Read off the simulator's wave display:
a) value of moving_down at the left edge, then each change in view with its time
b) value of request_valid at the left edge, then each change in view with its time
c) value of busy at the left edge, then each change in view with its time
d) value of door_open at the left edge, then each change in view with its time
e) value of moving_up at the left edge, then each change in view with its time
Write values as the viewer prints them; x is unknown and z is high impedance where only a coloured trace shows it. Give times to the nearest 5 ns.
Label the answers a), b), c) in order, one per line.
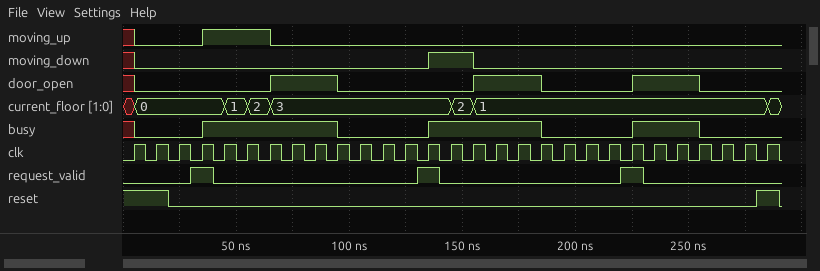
a) x, 0 at 5 ns, 1 at 135 ns, 0 at 155 ns
b) 0, 1 at 30 ns, 0 at 40 ns, 1 at 130 ns, 0 at 140 ns, 1 at 220 ns, 0 at 230 ns
c) x, 0 at 5 ns, 1 at 35 ns, 0 at 95 ns, 1 at 135 ns, 0 at 185 ns, 1 at 225 ns, 0 at 255 ns
d) x, 0 at 5 ns, 1 at 65 ns, 0 at 95 ns, 1 at 155 ns, 0 at 185 ns, 1 at 225 ns, 0 at 255 ns
e) x, 0 at 5 ns, 1 at 35 ns, 0 at 65 ns
